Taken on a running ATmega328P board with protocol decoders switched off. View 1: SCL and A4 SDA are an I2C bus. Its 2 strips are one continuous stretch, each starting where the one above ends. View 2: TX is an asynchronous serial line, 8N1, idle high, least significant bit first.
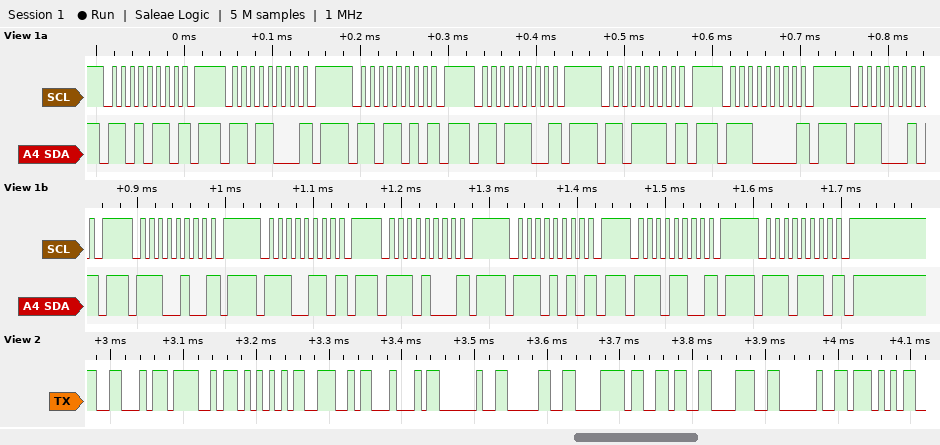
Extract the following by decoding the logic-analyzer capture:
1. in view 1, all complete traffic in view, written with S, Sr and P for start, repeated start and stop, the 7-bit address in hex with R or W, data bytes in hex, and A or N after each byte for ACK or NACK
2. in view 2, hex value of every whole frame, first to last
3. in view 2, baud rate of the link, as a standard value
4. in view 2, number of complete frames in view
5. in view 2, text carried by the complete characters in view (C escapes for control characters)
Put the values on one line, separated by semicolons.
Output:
S 6BW N P S 6CW N P S 6DW N P S 6EW N P S 6FW N P S 70W N P S 71W N P S 72W N P S 73W N P S 74W N P S 75W N P S 76W N P S 77W N P; 46 4F 55 4E 44 20 30 78 36 38 20 57; 115200 baud; 12; "FOUND 0x68 W"
